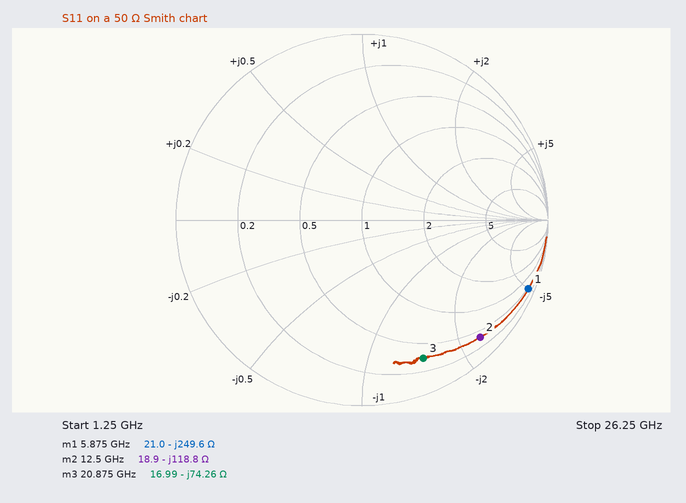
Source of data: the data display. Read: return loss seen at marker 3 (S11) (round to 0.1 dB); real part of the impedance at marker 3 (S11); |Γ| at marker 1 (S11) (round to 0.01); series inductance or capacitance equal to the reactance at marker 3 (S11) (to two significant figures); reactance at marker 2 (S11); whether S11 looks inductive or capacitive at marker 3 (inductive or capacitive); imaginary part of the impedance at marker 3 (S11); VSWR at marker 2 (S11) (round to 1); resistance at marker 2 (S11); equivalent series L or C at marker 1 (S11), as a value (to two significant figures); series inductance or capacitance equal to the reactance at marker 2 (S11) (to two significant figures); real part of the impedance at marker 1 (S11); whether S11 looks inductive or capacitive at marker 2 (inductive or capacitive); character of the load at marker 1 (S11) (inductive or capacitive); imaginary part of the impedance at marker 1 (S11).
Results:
1.8 dB
16.99 Ω
0.97
100 fF
-118.8 Ω
capacitive
-74.26 Ω
18
18.9 Ω
110 fF
110 fF
21.0 Ω
capacitive
capacitive
-249.6 Ω
